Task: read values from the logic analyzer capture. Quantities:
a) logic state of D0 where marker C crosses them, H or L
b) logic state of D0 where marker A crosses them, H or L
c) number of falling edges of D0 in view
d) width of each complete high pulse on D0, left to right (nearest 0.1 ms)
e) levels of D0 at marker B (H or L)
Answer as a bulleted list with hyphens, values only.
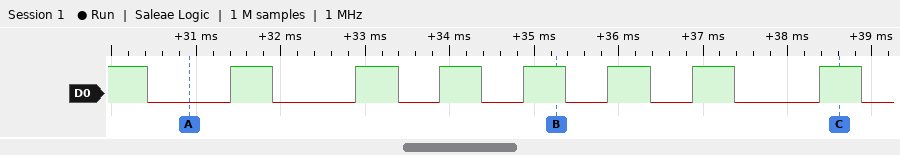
- D0=H
- D0=L
- 8
- 0.5 ms, 0.5 ms, 0.5 ms, 0.5 ms, 0.5 ms, 0.5 ms, 0.5 ms
- D0=H
